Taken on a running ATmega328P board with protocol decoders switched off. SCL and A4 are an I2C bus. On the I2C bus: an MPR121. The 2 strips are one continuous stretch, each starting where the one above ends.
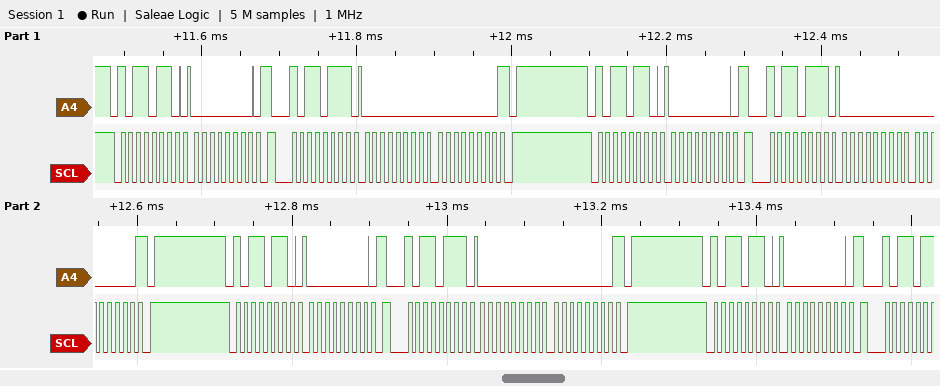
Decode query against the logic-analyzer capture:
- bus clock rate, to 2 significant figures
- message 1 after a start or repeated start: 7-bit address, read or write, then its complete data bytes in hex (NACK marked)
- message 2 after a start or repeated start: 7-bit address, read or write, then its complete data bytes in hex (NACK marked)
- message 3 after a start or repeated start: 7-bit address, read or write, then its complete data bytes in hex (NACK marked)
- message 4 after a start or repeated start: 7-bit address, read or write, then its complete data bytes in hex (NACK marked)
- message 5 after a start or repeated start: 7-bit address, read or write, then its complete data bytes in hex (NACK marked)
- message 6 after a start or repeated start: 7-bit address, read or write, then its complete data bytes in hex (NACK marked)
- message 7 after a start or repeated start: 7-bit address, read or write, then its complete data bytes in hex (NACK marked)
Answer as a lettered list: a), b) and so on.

a) 100 kHz
b) 0x5B write: 00
c) 0x5B read: 00 00 NACK
d) 0x5B write: 00
e) 0x5B read: 00 00 NACK
f) 0x5B write: 00
g) 0x5B read: 00 00 NACK
h) 0x5B write: 00
